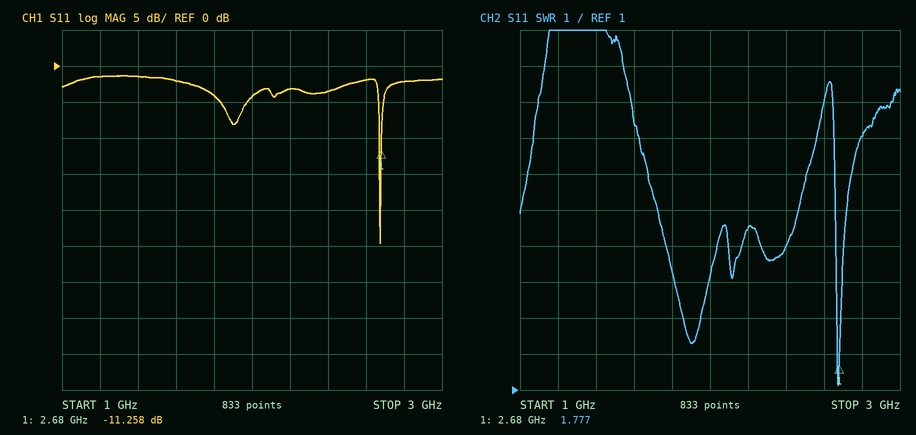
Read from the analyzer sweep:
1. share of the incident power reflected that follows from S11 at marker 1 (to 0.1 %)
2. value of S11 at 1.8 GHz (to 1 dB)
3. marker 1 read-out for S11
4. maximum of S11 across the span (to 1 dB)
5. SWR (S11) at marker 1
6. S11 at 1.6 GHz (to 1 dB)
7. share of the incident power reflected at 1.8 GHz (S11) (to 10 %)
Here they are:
7.5 %
-4 dB
-11.258 dB
-1 dB
1.777
-2 dB
40 %
